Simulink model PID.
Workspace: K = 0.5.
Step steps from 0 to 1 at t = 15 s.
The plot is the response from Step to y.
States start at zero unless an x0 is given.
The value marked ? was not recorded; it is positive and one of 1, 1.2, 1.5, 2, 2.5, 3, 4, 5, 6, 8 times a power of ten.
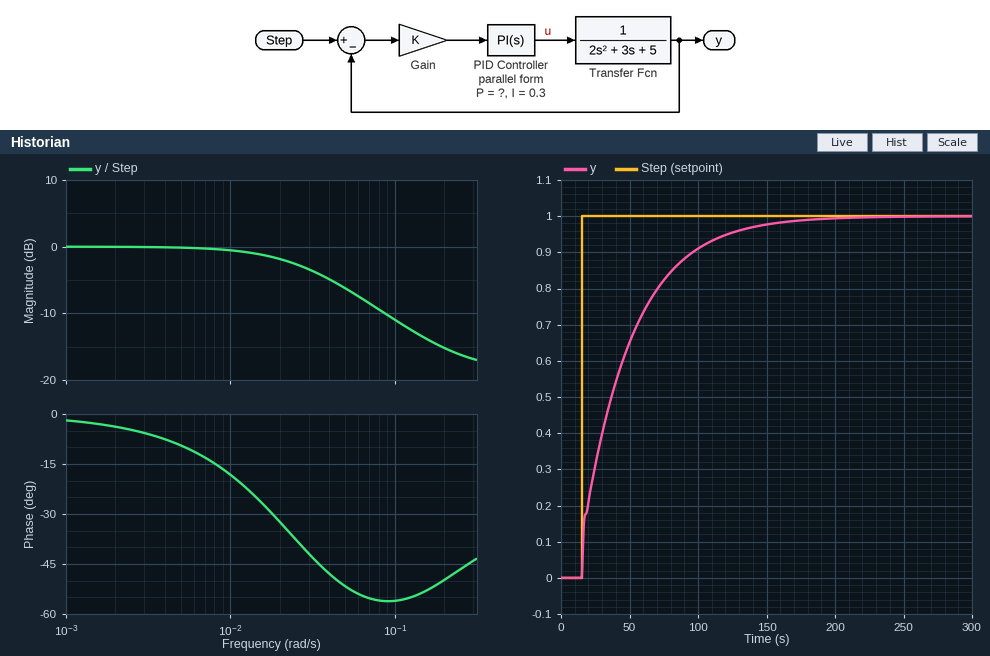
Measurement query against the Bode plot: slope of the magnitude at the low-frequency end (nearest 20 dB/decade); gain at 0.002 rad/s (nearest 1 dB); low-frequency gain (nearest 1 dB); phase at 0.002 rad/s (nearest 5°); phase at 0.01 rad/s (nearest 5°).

0 dB/decade
0 dB
0 dB
-5°
-20°
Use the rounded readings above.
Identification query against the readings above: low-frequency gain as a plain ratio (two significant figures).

1.0
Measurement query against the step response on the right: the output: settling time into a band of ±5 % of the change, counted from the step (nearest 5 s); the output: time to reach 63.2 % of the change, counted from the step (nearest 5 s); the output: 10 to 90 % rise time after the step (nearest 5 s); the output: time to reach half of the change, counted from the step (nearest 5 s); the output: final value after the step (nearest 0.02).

105 s
35 s
80 s
20 s
1.00
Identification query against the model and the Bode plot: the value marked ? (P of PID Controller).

1.2
